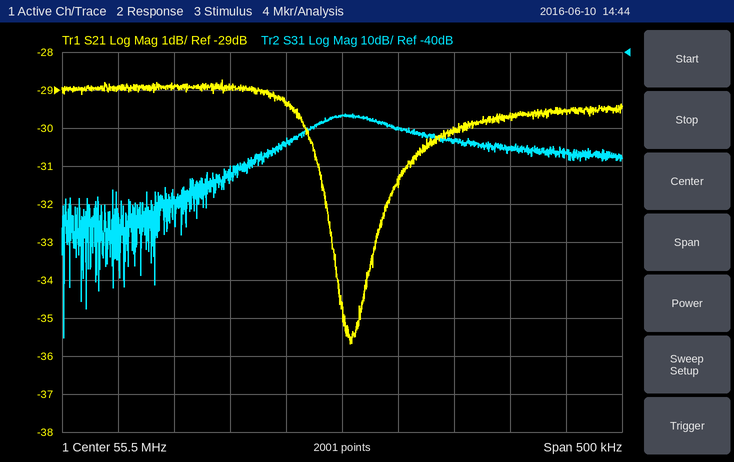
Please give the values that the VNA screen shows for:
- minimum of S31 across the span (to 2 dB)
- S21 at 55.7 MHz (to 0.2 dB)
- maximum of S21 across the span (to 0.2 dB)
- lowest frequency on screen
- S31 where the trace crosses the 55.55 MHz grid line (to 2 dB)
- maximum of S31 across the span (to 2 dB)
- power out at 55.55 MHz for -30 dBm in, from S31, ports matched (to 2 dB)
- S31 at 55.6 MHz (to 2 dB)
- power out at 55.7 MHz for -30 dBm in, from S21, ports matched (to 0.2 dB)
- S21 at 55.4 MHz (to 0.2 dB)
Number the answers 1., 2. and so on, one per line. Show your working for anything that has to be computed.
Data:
1. -116 dB
2. -29.6 dB
3. -28.8 dB
4. 55.25 MHz
5. -60 dB
6. -56 dB
7. -30 dBm + (-60 dB) = -90 dBm
8. -64 dB
9. -30 dBm + (-29.6 dB) = -59.6 dBm
10. -29.0 dB
